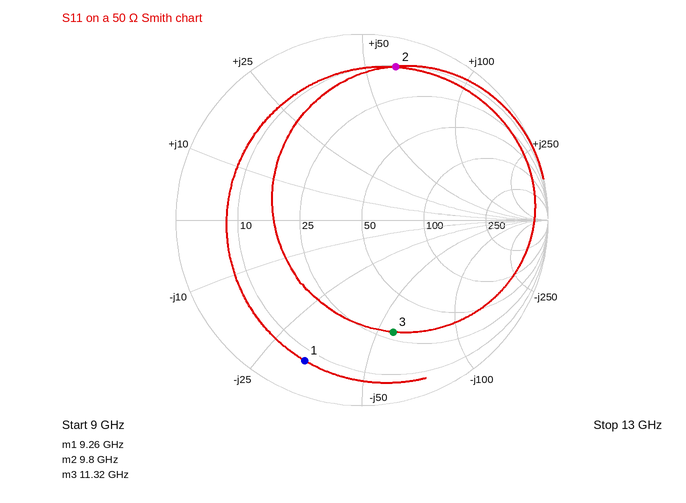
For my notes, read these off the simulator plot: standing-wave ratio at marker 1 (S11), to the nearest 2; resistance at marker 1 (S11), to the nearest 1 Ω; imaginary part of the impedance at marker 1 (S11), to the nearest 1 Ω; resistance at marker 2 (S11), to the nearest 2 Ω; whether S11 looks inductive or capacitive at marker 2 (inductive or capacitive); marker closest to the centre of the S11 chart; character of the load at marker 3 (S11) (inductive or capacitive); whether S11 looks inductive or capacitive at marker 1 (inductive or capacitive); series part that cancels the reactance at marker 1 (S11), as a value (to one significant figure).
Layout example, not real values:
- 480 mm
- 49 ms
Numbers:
- 10
- 7 Ω
- -33 Ω
- 10 Ω
- inductive
- marker 3
- capacitive
- capacitive
- 600 pH
